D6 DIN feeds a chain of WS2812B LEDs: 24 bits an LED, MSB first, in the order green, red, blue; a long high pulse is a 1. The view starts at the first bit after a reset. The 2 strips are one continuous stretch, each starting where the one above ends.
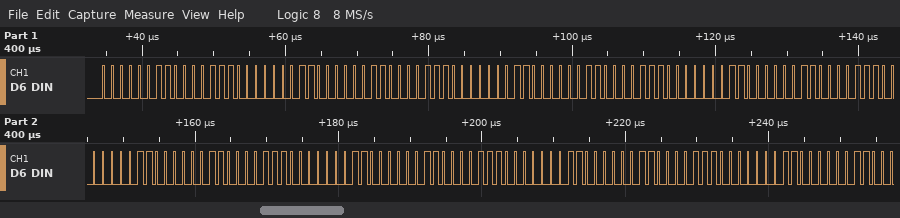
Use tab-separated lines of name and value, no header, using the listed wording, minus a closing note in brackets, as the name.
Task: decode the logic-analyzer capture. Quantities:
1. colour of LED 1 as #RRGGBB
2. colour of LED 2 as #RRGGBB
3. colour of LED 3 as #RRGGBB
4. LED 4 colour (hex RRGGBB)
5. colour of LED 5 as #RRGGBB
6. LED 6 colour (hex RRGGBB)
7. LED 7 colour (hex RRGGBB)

colour of LED 1 as #RRGGBB	#0E0303
colour of LED 2 as #RRGGBB	#0E0303
colour of LED 3 as #RRGGBB	#0E0303
LED 4 colour	#0E0303
colour of LED 5 as #RRGGBB	#0E0303
LED 6 colour	#0E0303
LED 7 colour	#0E0303
